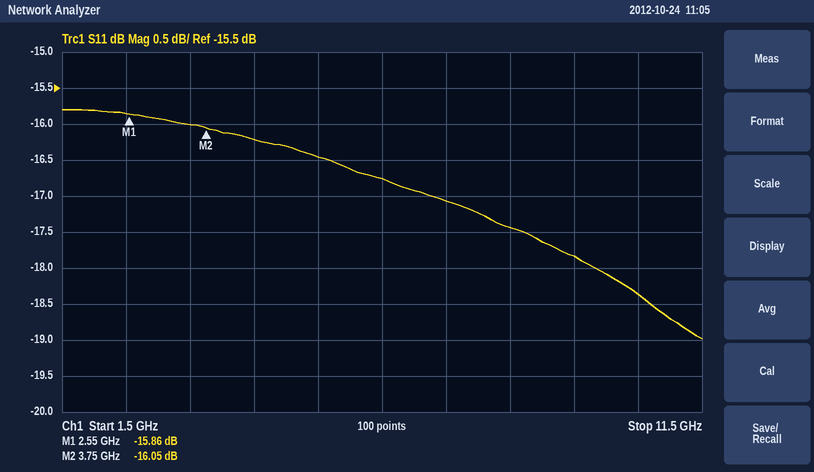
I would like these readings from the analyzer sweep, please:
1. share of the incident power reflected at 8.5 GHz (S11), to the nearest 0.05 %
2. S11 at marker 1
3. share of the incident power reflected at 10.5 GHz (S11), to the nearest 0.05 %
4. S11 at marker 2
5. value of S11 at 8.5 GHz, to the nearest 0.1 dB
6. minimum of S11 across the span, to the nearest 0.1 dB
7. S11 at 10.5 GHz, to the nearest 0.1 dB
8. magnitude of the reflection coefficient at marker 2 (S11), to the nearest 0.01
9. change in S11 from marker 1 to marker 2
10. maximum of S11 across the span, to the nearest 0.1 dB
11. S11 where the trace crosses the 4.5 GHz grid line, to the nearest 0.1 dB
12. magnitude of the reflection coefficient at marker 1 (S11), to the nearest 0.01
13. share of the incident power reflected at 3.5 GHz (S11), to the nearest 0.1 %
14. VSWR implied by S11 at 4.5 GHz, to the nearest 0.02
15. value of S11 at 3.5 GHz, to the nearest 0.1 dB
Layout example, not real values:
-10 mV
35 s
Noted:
1.80 %
-15.86 dB
1.45 %
-16.05 dB
-17.4 dB
-19.0 dB
-18.4 dB
0.16
-0.19 dB
-15.8 dB
-16.2 dB
0.16
2.5 %
1.36
-16.0 dB
